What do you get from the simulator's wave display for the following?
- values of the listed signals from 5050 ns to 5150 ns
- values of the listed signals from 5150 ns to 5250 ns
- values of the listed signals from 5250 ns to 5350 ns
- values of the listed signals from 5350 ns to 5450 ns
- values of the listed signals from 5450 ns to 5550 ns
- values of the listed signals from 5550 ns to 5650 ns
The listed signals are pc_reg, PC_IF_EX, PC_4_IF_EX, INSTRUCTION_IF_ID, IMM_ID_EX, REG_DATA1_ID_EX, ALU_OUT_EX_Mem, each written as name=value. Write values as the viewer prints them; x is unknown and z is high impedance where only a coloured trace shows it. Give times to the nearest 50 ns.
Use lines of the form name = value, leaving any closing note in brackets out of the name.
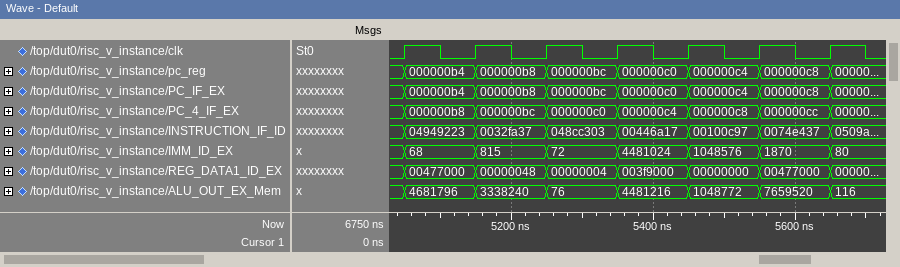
values of the listed signals from 5050 ns to 5150 ns = pc_reg=000000b4, PC_IF_EX=000000b4, PC_4_IF_EX=000000b8, INSTRUCTION_IF_ID=04949223, IMM_ID_EX=68, REG_DATA1_ID_EX=00477000, ALU_OUT_EX_Mem=4681796
values of the listed signals from 5150 ns to 5250 ns = pc_reg=000000b8, PC_IF_EX=000000b8, PC_4_IF_EX=000000bc, INSTRUCTION_IF_ID=0032fa37, IMM_ID_EX=815, REG_DATA1_ID_EX=00000048, ALU_OUT_EX_Mem=3338240
values of the listed signals from 5250 ns to 5350 ns = pc_reg=000000bc, PC_IF_EX=000000bc, PC_4_IF_EX=000000c0, INSTRUCTION_IF_ID=048cc303, IMM_ID_EX=72, REG_DATA1_ID_EX=00000004, ALU_OUT_EX_Mem=76
values of the listed signals from 5350 ns to 5450 ns = pc_reg=000000c0, PC_IF_EX=000000c0, PC_4_IF_EX=000000c4, INSTRUCTION_IF_ID=00446a17, IMM_ID_EX=4481024, REG_DATA1_ID_EX=003f9000, ALU_OUT_EX_Mem=4481216
values of the listed signals from 5450 ns to 5550 ns = pc_reg=000000c4, PC_IF_EX=000000c4, PC_4_IF_EX=000000c8, INSTRUCTION_IF_ID=00100c97, IMM_ID_EX=1048576, REG_DATA1_ID_EX=00000000, ALU_OUT_EX_Mem=1048772
values of the listed signals from 5550 ns to 5650 ns = pc_reg=000000c8, PC_IF_EX=000000c8, PC_4_IF_EX=000000cc, INSTRUCTION_IF_ID=0074e437, IMM_ID_EX=1870, REG_DATA1_ID_EX=00477000, ALU_OUT_EX_Mem=7659520
